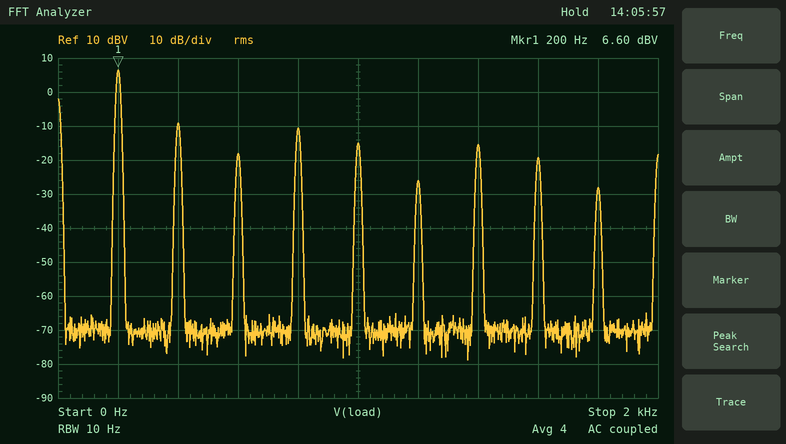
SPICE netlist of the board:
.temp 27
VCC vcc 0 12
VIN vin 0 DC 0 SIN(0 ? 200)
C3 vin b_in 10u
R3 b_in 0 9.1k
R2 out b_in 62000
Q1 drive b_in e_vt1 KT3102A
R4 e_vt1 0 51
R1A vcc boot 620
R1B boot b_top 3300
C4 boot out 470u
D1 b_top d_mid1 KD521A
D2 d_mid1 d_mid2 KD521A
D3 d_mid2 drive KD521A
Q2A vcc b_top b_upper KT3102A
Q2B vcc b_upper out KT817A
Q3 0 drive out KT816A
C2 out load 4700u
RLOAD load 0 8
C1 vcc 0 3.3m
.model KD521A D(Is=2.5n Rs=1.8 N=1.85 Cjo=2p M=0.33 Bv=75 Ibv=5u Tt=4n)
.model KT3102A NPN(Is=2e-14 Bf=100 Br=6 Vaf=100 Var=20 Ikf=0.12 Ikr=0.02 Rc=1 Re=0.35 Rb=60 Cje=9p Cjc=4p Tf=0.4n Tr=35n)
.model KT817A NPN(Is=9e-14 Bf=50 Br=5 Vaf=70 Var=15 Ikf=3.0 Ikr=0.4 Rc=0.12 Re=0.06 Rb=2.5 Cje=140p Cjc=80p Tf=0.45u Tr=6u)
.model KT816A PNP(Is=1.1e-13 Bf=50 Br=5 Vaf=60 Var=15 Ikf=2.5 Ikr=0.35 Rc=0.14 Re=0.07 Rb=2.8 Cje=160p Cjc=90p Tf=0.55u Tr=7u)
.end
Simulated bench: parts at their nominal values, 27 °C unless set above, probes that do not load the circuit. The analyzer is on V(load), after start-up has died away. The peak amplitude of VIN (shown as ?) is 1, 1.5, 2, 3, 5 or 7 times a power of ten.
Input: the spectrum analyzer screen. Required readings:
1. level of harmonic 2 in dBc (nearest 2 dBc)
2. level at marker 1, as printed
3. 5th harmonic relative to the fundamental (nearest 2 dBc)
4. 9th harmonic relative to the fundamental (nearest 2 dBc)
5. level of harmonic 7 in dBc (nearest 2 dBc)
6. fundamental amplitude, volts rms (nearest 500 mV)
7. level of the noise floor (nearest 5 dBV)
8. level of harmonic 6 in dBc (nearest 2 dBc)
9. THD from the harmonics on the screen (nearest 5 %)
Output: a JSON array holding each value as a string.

["-16 dBc", "6.60 dBV", "-22 dBc", "-34 dBc", "-22 dBc", "2.0 V", "-70 dBV", "-32 dBc", "25 %"]
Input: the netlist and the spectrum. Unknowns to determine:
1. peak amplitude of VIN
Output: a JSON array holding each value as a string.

["300 mV"]
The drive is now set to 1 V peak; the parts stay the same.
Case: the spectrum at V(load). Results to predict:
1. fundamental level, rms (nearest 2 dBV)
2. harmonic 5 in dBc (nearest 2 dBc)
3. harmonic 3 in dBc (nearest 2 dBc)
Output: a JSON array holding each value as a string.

["10 dBV", "-24 dBc", "-18 dBc"]
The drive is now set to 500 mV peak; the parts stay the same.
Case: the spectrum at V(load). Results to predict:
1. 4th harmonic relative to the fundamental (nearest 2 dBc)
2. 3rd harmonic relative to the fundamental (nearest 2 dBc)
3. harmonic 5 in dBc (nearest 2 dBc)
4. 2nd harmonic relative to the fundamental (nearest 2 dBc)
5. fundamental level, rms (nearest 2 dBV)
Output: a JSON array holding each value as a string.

["-24 dBc", "-16 dBc", "-24 dBc", "-24 dBc", "8 dBV"]
